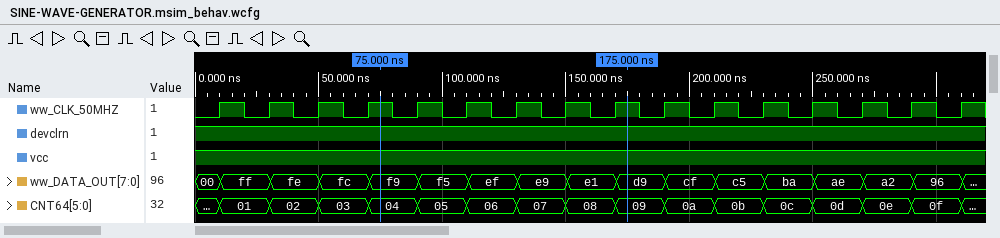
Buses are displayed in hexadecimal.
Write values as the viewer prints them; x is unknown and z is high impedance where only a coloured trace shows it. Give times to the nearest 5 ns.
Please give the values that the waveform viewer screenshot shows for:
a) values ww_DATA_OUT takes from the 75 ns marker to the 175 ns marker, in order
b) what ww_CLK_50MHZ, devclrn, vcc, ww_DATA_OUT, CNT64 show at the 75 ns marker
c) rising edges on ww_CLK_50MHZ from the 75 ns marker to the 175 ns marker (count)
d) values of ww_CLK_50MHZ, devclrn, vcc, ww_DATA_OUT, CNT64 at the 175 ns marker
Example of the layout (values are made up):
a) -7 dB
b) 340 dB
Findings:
a) f9, f5, ef, e9, e1, d9
b) ww_CLK_50MHZ=1, devclrn=1, vcc=1, ww_DATA_OUT=f9, CNT64=04
c) 5
d) ww_CLK_50MHZ=1, devclrn=1, vcc=1, ww_DATA_OUT=d9, CNT64=09
